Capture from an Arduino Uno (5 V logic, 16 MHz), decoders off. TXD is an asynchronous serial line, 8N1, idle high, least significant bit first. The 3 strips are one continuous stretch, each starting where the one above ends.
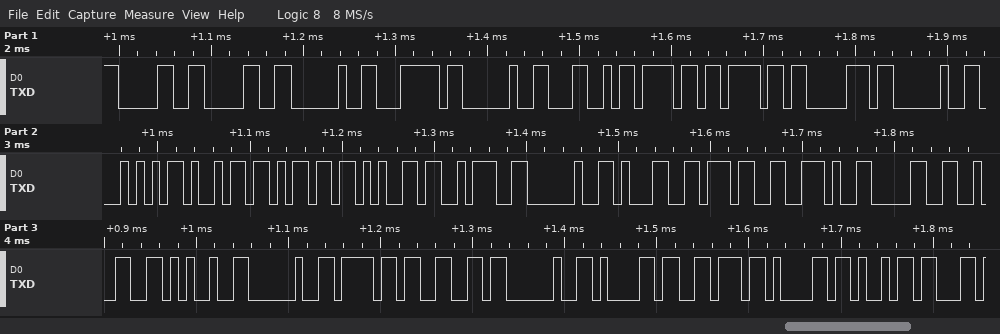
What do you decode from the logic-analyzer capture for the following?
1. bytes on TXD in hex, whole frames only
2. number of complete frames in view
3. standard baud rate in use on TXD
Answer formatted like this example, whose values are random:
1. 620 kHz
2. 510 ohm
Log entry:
1. 30 30 20 7C 20 4C 6F 6F 70 20 54 69 6D 65 3A 20 31 37 2E 30 32 25 20 6F 66 20 61 76 61 69
2. 30
3. 115200 baud
